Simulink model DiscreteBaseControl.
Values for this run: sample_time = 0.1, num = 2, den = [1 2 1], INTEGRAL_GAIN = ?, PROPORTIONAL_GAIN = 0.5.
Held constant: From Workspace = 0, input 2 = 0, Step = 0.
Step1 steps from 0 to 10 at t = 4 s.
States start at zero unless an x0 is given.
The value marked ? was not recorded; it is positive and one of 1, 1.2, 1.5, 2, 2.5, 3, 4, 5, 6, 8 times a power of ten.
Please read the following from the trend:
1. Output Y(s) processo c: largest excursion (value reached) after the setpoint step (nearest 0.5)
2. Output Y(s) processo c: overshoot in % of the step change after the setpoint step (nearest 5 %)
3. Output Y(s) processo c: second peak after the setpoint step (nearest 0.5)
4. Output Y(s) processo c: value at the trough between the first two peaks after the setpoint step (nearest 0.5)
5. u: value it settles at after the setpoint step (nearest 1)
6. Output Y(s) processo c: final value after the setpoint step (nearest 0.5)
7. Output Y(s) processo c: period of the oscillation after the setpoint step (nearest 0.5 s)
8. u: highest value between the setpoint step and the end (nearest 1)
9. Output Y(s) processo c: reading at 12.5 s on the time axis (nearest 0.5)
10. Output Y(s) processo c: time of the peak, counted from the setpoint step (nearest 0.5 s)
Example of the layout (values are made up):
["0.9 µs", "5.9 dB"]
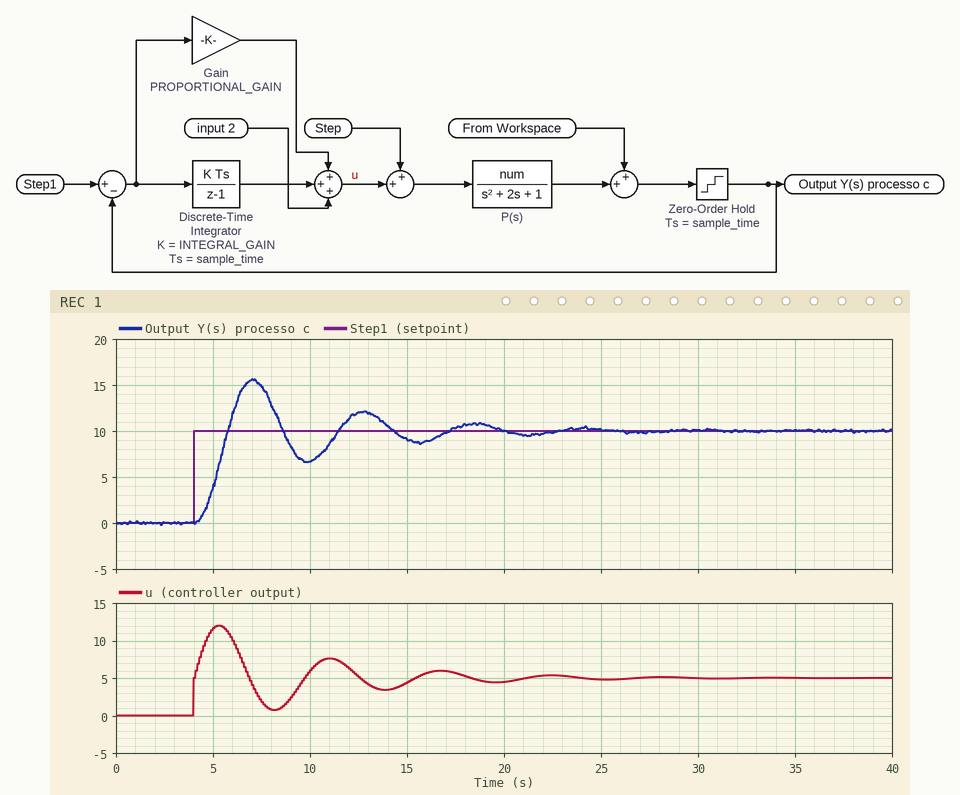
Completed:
["15.5", "55 %", "12.0", "6.5", "5", "10.0", "5.5 s", "12", "12.0", "3.0 s"]
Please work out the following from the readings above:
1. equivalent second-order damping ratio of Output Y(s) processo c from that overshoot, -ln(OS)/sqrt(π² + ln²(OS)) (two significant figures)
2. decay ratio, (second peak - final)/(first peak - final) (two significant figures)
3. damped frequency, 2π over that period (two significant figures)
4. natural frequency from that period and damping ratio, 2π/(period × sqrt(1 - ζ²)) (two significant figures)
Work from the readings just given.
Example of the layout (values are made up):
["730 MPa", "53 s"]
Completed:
["0.19", "0.36", "1.1 rad/s", "1.2 rad/s"]
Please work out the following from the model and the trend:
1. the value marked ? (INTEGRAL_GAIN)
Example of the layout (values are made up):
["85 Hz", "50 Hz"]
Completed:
["1"]
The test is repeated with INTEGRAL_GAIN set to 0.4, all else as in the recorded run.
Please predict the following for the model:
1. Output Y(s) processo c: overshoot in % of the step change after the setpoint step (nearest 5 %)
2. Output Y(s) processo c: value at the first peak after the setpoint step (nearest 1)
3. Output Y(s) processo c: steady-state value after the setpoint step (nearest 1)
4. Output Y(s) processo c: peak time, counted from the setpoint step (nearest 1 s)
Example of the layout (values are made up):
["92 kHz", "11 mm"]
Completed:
["10 %", "11", "10", "4 s"]
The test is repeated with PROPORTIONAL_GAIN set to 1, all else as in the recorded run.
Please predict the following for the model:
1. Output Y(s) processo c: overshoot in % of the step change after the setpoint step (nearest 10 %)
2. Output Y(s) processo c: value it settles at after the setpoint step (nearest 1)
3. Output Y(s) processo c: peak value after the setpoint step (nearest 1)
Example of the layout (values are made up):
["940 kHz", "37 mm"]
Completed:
["40 %", "10", "14"]
